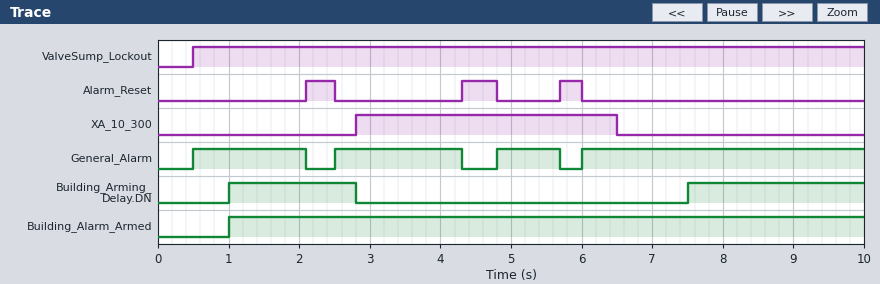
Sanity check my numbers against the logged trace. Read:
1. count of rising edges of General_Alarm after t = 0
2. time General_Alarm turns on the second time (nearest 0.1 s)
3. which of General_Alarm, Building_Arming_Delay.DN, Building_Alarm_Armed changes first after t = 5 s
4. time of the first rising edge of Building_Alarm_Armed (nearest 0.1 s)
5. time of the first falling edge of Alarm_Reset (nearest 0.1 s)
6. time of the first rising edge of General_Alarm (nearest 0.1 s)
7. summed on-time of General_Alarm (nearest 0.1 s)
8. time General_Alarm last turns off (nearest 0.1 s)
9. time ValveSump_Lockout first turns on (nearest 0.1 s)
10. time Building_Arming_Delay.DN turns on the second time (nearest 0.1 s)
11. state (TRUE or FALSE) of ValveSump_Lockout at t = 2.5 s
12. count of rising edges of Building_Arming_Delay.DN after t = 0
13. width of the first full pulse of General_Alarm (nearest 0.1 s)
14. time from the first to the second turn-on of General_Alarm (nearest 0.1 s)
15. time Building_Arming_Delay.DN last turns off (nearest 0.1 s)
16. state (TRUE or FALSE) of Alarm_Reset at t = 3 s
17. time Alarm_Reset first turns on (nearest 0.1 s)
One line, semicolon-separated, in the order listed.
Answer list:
4; 2.5 s; General_Alarm; 1.0 s; 2.5 s; 0.5 s; 8.3 s; 5.7 s; 0.5 s; 7.5 s; TRUE; 2; 1.6 s; 2.0 s; 2.8 s; FALSE; 2.1 s
